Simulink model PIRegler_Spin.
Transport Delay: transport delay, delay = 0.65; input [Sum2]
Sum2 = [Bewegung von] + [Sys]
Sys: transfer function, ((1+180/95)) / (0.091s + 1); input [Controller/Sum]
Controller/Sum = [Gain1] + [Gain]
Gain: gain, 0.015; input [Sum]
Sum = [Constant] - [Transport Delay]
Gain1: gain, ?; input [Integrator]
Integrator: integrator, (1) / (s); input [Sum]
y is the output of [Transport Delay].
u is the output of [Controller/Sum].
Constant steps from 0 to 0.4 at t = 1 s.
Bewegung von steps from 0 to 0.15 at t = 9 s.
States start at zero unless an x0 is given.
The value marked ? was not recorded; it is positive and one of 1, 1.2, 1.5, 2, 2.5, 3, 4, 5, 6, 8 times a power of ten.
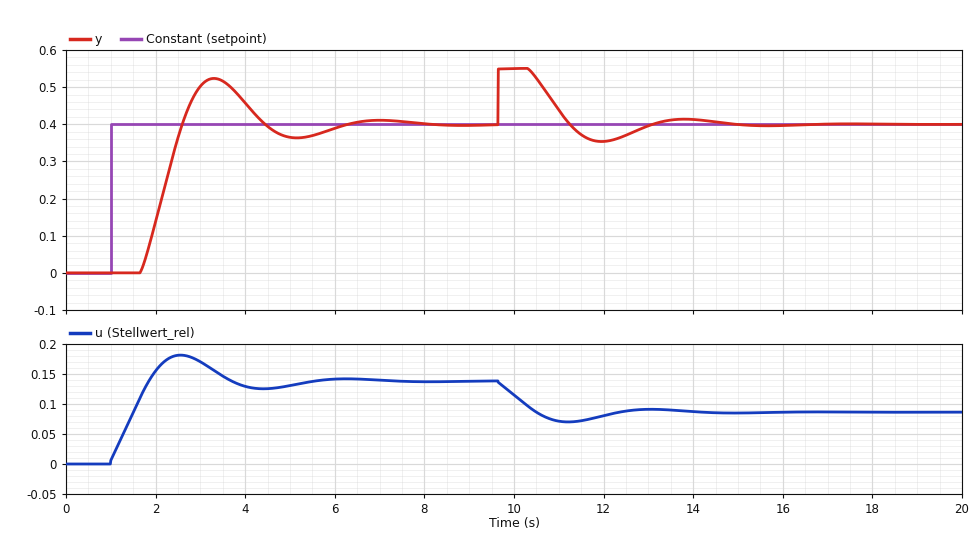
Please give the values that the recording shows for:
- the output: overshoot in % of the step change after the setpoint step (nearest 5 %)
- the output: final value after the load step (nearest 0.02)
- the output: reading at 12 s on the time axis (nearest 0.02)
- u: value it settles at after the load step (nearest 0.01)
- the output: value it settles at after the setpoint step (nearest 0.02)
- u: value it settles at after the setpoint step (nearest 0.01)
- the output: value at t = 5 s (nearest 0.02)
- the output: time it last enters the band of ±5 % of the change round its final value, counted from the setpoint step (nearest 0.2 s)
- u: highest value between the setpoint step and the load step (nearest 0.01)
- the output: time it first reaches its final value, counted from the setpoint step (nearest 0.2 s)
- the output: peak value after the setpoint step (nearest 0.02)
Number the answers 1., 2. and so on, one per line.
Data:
1. 30 %
2. 0.40
3. 0.36
4. 0.09
5. 0.40
6. 0.14
7. 0.36
8. 4.8 s
9. 0.18
10. 1.6 s
11. 0.52
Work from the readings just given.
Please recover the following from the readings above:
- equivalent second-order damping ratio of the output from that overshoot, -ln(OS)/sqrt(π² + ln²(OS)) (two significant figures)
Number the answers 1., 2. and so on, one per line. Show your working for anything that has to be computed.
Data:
1. ln(0.3) = -1.204; 1.204 / sqrt(9.870 + 1.450) = 0.36
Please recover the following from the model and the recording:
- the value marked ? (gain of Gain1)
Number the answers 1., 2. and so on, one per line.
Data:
1. 0.4
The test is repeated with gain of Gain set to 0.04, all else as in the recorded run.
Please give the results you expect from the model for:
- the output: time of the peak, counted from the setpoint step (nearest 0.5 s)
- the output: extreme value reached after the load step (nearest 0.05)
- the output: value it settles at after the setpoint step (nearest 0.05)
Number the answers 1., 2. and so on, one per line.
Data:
1. 2.0 s
2. 0.55
3. 0.40
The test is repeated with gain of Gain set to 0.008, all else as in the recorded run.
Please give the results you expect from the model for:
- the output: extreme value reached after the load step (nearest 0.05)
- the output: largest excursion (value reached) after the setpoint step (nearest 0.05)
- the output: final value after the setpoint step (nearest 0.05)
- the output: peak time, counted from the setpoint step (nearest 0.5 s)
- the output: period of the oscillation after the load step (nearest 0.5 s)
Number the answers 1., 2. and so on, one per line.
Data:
1. 0.55
2. 0.55
3. 0.40
4. 2.5 s
5. 3.5 s
